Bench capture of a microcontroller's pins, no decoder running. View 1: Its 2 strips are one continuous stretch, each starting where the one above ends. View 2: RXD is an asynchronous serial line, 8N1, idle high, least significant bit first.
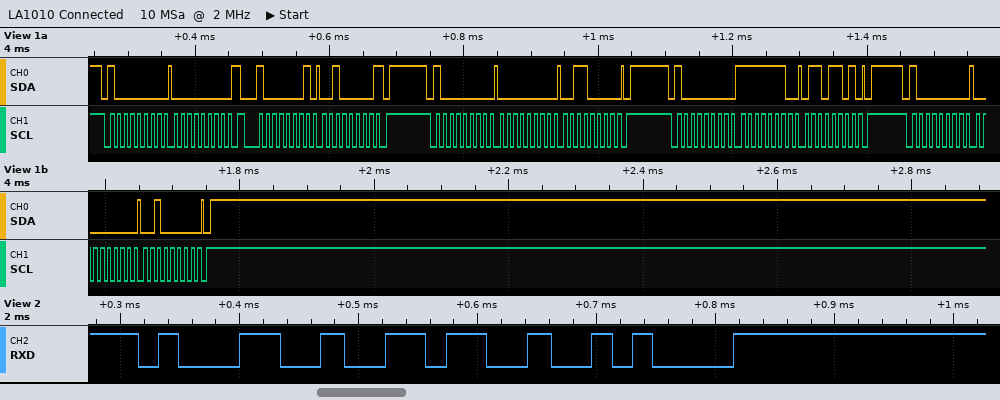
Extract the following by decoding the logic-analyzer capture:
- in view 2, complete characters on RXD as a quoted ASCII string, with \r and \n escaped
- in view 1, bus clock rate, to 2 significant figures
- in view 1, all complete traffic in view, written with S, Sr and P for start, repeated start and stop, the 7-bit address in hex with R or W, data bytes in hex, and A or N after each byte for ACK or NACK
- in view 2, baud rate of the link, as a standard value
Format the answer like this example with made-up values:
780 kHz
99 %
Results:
"16\n"
100 kHz
S 40W A 00 A Sr 40R A 20 N P S 40W A 00 A 30 A P S 40W A FE A 6D A P S 40W A 00 A 20 A P
57600 baud
